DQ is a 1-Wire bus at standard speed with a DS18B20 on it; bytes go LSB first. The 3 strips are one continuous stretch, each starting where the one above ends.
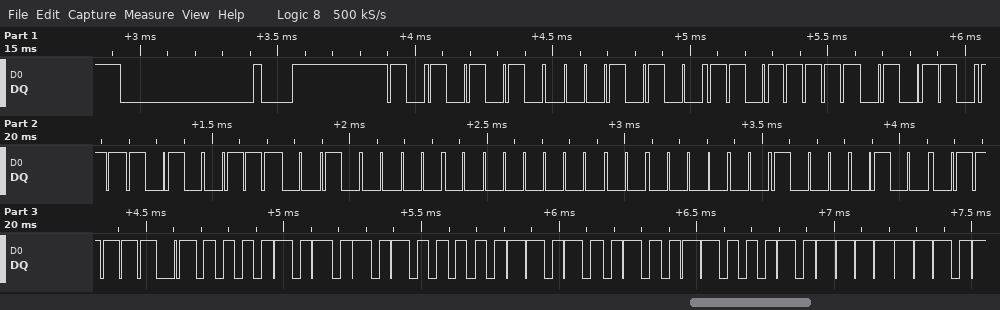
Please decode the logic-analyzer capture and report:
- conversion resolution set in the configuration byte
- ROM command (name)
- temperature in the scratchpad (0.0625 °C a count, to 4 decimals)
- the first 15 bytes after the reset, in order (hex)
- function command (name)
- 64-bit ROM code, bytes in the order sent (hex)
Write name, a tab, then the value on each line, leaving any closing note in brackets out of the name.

conversion resolution set in the configuration byte	12 bits
ROM command	Match ROM
temperature in the scratchpad	85.0000 °C
the first 15 bytes after the reset, in order	55 28 FB DA E5 04 00 00 21 BE 50 05 4B 46 7F
function command	Read Scratchpad
64-bit ROM code, bytes in the order sent	28 FB DA E5 04 00 00 21
